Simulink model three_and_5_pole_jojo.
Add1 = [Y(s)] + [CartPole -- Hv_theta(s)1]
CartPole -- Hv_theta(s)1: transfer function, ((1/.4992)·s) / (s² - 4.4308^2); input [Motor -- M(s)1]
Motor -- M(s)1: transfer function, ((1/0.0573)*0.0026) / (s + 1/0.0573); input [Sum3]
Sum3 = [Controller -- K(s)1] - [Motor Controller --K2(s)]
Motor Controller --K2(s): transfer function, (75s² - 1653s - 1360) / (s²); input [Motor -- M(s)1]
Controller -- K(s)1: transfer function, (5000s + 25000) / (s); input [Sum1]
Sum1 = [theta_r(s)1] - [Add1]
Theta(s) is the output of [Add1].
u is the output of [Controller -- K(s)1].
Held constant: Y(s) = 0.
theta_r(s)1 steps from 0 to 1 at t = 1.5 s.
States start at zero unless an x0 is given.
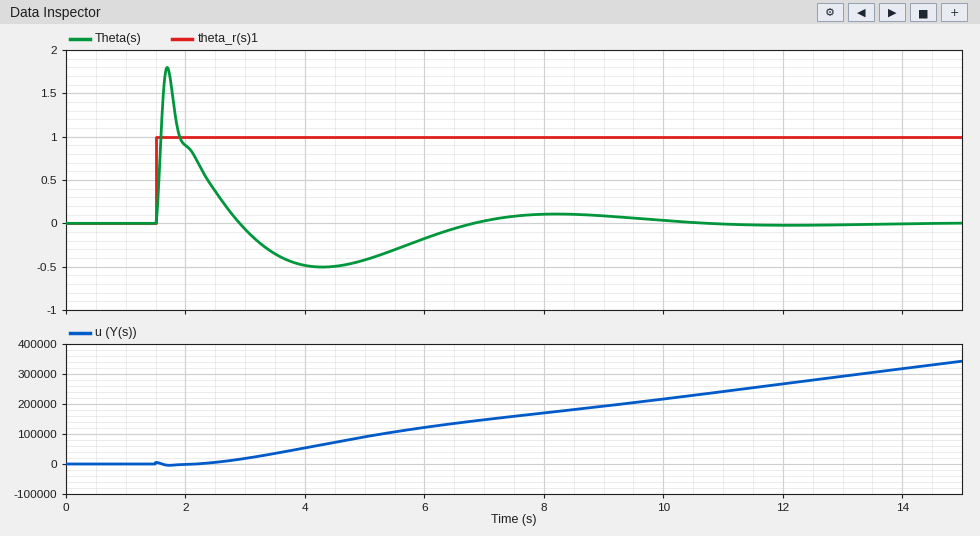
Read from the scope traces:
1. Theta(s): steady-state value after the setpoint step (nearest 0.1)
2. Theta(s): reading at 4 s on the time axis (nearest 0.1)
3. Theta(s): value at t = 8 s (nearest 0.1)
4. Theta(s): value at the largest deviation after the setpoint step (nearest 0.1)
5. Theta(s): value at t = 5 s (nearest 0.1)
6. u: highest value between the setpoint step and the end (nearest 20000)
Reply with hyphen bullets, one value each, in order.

- 0.0
- -0.5
- 0.1
- 1.8
- -0.4
- 340000
